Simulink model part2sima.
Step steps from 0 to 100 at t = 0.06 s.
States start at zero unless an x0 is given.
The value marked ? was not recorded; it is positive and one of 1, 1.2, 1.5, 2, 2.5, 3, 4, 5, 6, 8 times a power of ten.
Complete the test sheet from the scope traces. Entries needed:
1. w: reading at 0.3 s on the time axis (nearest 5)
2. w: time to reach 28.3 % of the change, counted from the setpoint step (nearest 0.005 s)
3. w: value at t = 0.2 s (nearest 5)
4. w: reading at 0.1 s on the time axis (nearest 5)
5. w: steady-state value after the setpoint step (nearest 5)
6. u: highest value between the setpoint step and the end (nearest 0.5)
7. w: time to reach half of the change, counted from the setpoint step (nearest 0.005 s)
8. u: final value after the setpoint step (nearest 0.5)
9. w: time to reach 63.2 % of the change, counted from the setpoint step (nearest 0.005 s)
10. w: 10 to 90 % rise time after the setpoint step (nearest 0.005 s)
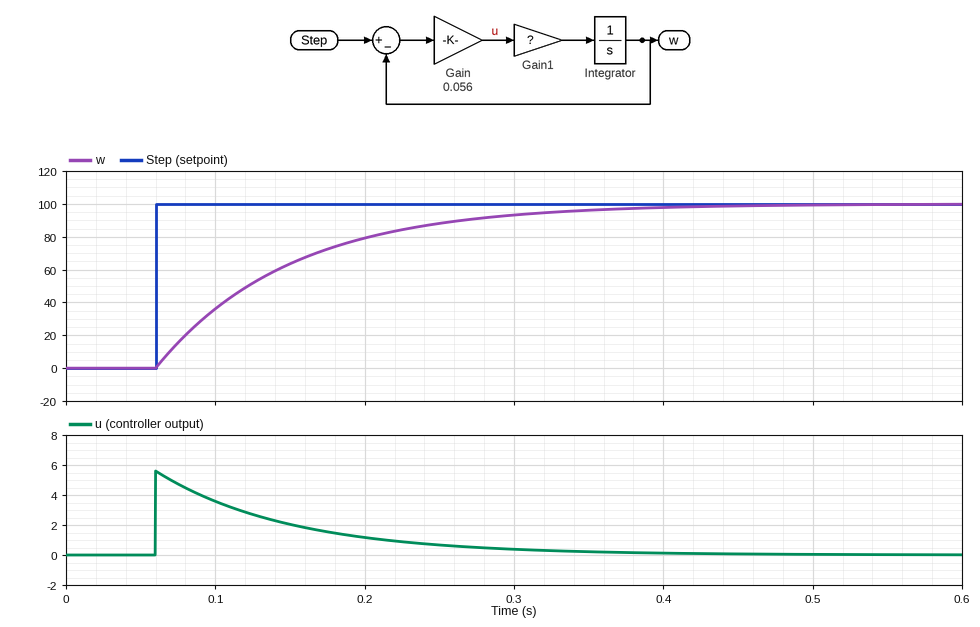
95
0.030 s
80
35
100
5.5
0.060 s
0.0
0.090 s
0.195 s
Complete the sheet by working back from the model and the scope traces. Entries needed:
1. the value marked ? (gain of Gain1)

200
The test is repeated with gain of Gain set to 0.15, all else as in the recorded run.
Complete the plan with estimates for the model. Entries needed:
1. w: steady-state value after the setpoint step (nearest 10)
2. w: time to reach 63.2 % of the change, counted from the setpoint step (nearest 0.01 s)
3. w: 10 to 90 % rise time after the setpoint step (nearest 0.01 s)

100
0.03 s
0.07 s
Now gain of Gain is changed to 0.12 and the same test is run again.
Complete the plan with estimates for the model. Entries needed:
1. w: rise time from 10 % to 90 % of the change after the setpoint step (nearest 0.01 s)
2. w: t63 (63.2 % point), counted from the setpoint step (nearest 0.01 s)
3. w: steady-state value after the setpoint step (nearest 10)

0.09 s
0.04 s
100
